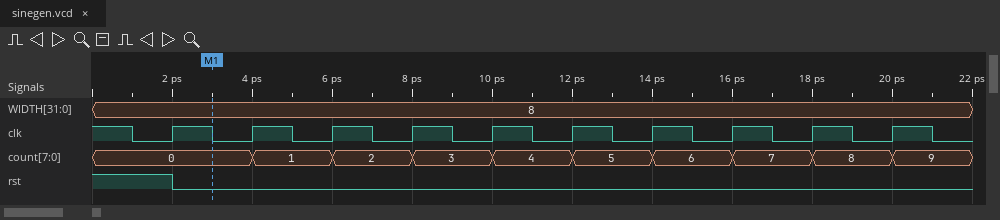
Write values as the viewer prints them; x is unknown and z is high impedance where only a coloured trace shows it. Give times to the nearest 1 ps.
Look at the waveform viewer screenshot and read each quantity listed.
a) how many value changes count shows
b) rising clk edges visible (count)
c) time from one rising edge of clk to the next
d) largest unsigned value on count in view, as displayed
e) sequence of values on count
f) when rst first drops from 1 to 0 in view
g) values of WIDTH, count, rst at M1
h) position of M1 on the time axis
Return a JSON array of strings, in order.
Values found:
["9", "10", "2 ps", "9", "0, 1, 2, 3, 4, 5, 6, 7, 8, 9", "2 ps", "WIDTH=8, count=0, rst=0", "3 ps"]
